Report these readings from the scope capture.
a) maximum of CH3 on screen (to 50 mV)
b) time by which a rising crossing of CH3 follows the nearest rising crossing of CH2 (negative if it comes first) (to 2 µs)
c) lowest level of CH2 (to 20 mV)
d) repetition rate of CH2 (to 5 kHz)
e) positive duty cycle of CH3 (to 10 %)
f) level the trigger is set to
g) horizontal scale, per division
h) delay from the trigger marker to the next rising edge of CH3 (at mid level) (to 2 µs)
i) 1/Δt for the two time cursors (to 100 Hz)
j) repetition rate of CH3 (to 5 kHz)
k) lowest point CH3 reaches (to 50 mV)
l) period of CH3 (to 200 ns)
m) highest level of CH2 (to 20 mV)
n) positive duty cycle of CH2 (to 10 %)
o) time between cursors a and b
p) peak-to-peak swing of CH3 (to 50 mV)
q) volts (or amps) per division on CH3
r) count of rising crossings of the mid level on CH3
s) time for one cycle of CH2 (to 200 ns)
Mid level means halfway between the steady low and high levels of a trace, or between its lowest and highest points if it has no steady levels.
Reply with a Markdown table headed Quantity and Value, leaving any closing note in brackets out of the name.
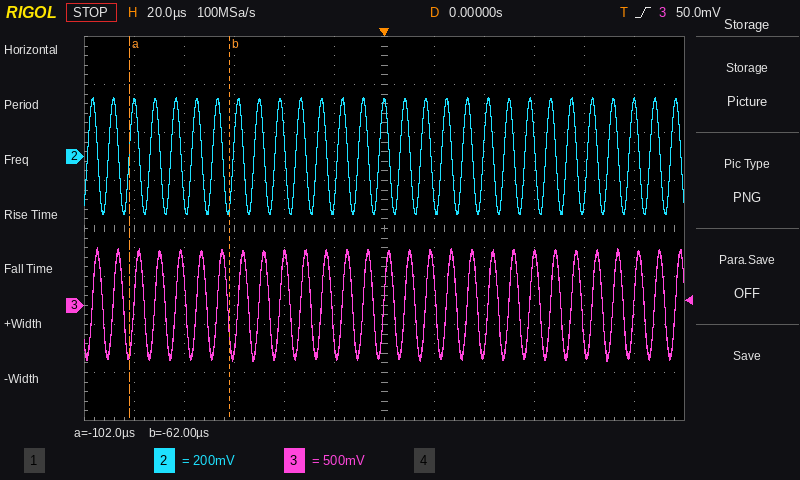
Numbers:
| Quantity | Value |
|---|---|
| maximum of CH3 on screen | 600 mV |
| time by which a rising crossing of CH3 follows the nearest rising crossing of CH2 (negative if it comes first) | +2 µs |
| lowest level of CH2 | -240 mV |
| repetition rate of CH2 | 120 kHz |
| positive duty cycle of CH3 | 50 % |
| level the trigger is set to | 50.0 mV |
| horizontal scale, per division | 20 µs |
| delay from the trigger marker to the next rising edge of CH3 (at mid level) | 8 µs |
| 1/Δt for the two time cursors | 25.0 kHz |
| repetition rate of CH3 | 120 kHz |
| lowest point CH3 reaches | -600 mV |
| period of CH3 | 8.4 µs |
| highest level of CH2 | 240 mV |
| positive duty cycle of CH2 | 50 % |
| time between cursors a and b | 40 µs |
| peak-to-peak swing of CH3 | 1.20 V |
| volts (or amps) per division on CH3 | 500 mV |
| count of rising crossings of the mid level on CH3 | 29 |
| time for one cycle of CH2 | 8.4 µs |
